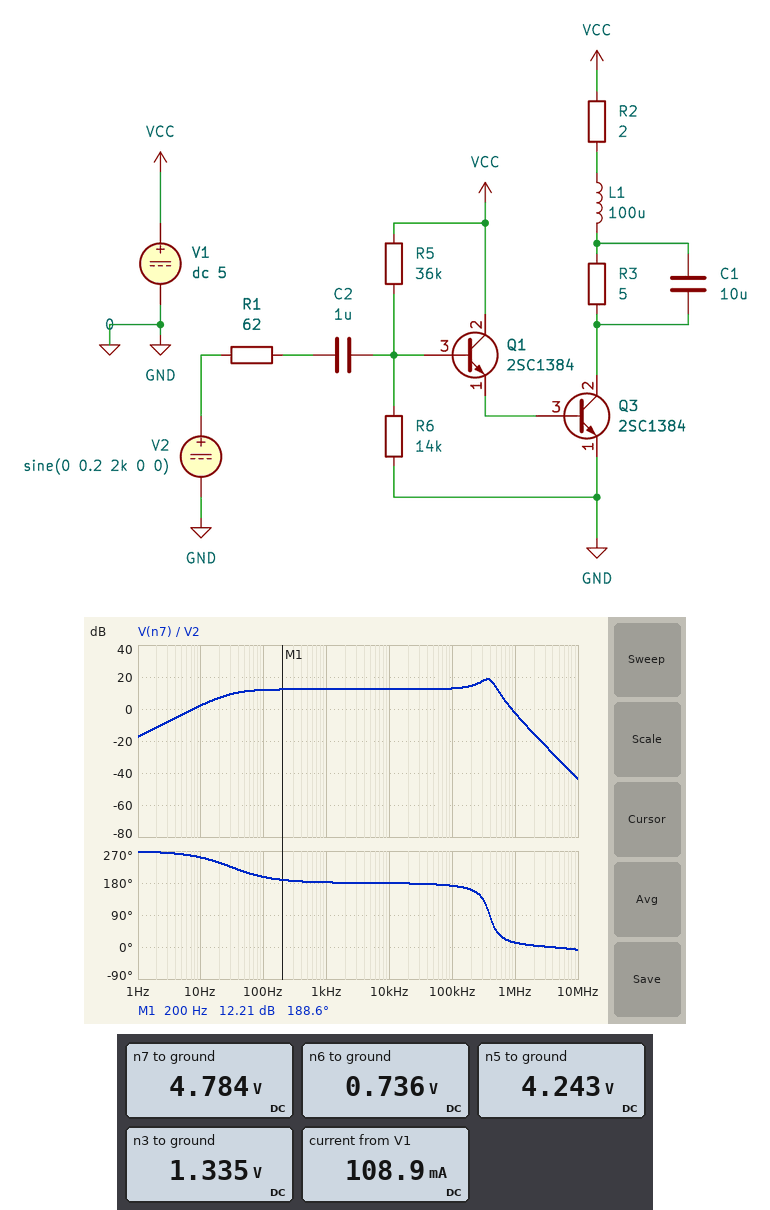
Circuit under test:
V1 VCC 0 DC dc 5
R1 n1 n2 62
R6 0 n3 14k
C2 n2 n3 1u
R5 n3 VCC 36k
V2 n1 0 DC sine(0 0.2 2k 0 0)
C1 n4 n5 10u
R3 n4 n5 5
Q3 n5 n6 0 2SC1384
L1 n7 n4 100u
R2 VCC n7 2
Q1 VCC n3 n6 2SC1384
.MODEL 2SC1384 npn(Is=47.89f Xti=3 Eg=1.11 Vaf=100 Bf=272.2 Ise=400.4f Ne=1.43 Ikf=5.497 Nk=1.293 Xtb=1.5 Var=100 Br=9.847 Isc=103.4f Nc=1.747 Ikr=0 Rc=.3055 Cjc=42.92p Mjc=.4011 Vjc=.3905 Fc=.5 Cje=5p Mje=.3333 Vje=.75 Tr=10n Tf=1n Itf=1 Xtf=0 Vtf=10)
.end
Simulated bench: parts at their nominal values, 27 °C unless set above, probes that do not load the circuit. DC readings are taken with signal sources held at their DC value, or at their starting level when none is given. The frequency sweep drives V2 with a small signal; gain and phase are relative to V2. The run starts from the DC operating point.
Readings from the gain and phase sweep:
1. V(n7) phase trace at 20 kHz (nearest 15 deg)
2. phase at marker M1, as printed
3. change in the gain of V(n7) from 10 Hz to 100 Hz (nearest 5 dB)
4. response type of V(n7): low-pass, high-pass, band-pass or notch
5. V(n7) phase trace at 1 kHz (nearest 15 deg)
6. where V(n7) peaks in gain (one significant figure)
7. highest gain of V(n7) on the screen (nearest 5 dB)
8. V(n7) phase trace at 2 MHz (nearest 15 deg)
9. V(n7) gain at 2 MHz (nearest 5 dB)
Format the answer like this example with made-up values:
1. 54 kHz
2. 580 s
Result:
1. 180 deg
2. 188.6 deg
3. 10 dB
4. band-pass
5. 180 deg
6. 400 kHz
7. 20 dB
8. 0 deg
9. -15 dB
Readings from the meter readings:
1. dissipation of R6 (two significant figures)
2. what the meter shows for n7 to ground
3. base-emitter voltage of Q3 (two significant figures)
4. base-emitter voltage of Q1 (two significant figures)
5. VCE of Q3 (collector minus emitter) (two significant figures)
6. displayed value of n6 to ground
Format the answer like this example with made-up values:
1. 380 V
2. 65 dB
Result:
1. 130 µW
2. 4.784 V
3. 740 mV
4. 600 mV
5. 4.2 V
6. 0.736 V
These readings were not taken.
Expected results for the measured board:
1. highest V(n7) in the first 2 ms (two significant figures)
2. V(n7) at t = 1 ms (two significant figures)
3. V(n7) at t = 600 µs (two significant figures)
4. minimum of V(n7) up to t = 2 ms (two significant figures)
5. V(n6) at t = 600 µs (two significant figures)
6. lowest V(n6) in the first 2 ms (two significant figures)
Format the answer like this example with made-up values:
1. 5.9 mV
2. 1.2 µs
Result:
1. 5.0 V
2. 4.9 V
3. 3.2 V
4. 3.1 V
5. 810 mV
6. 610 mV
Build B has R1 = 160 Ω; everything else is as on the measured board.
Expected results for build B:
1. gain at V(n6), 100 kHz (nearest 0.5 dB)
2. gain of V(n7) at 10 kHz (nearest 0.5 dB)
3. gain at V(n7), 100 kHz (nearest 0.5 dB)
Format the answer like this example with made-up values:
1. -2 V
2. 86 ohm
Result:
1. -5.5 dB
2. 12.0 dB
3. 12.5 dB
